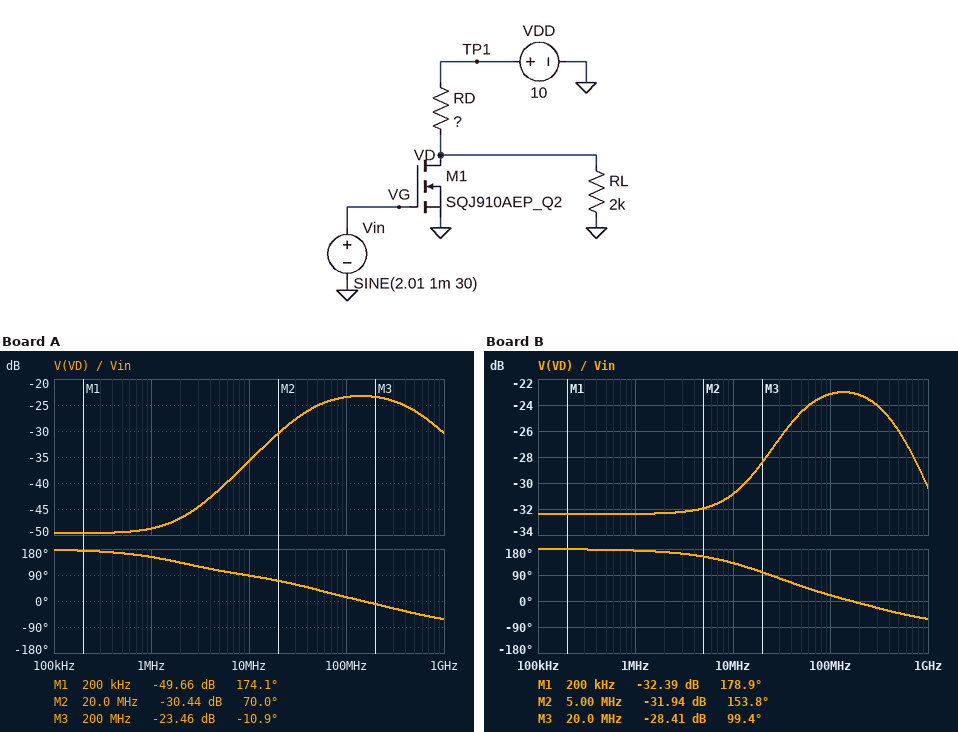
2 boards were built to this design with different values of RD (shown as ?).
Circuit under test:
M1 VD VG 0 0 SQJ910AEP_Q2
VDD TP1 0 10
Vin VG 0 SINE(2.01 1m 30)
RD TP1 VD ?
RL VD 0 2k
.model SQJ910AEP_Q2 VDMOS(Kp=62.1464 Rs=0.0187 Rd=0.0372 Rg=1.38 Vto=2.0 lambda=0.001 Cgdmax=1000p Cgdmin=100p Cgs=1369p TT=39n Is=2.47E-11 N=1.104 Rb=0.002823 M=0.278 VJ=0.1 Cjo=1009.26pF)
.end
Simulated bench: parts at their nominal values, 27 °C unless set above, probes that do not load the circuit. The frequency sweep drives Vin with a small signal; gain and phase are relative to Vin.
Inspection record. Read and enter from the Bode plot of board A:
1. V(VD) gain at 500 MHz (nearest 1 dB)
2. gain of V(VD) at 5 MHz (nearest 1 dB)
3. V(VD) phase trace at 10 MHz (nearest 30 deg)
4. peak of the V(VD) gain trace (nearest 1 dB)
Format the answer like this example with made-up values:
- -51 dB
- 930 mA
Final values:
- -26 dB
- -41 dB
- 90 deg
- -23 dB
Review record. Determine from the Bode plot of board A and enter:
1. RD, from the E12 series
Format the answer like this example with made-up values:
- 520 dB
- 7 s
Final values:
- 4.7 kΩ
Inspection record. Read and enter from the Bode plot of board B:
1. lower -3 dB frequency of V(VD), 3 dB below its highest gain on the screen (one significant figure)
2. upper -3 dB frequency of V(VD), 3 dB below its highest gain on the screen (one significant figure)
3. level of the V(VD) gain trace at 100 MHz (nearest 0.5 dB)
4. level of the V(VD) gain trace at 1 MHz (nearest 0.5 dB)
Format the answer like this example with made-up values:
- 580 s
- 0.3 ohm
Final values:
- 30 MHz
- 500 MHz
- -23.0 dB
- -32.5 dB
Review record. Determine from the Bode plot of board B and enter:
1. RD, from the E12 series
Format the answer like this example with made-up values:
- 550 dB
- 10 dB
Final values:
- 680 Ω
